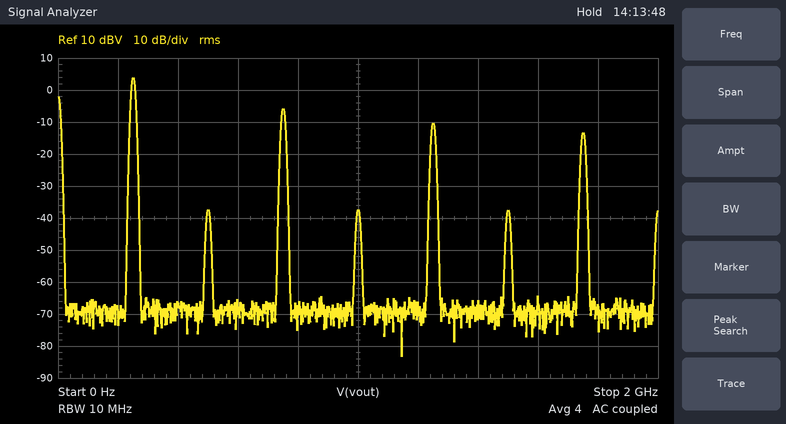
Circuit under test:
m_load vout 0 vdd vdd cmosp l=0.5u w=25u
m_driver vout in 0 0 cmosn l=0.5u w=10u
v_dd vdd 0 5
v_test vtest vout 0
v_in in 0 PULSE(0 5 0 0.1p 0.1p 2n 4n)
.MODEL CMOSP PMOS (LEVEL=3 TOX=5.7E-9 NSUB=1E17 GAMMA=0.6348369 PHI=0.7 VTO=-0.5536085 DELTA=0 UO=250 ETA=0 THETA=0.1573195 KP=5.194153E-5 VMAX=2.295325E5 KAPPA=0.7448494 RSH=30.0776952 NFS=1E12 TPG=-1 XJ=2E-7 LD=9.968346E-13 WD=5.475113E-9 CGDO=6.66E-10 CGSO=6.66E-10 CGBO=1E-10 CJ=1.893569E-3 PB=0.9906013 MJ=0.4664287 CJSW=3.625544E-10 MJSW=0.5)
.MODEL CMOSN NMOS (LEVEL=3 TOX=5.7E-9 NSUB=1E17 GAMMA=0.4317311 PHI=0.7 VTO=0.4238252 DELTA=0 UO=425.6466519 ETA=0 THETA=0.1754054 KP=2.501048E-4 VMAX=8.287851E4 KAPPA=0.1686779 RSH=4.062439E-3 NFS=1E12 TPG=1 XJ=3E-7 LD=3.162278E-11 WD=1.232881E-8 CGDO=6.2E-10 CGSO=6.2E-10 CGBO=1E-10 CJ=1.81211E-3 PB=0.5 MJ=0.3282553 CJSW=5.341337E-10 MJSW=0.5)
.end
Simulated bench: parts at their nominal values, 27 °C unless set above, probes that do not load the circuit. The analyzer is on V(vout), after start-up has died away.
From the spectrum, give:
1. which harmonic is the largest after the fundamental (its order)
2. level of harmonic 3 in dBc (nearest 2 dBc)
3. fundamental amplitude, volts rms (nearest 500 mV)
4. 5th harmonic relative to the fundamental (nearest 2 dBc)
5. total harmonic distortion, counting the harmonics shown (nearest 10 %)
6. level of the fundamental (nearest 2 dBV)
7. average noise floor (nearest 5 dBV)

3
-10 dBc
1.5 V
-14 dBc
40 %
4 dBV
-70 dBV
